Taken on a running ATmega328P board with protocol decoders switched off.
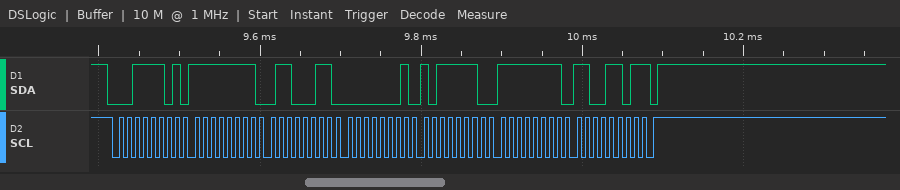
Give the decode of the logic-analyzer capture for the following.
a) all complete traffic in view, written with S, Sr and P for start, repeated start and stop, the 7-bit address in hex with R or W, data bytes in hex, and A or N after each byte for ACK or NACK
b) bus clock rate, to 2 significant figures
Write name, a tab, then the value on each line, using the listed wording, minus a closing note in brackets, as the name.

all complete traffic in view, written with S, Sr and P for start, repeated start and stop, the 7-bit address in hex with R or W, data bytes in hex, and A or N after each byte for ACK or NACK	S 1ER A FF A 63 A 01 A BE A FF A CD N P
bus clock rate, to 2 significant figures	100 kHz
